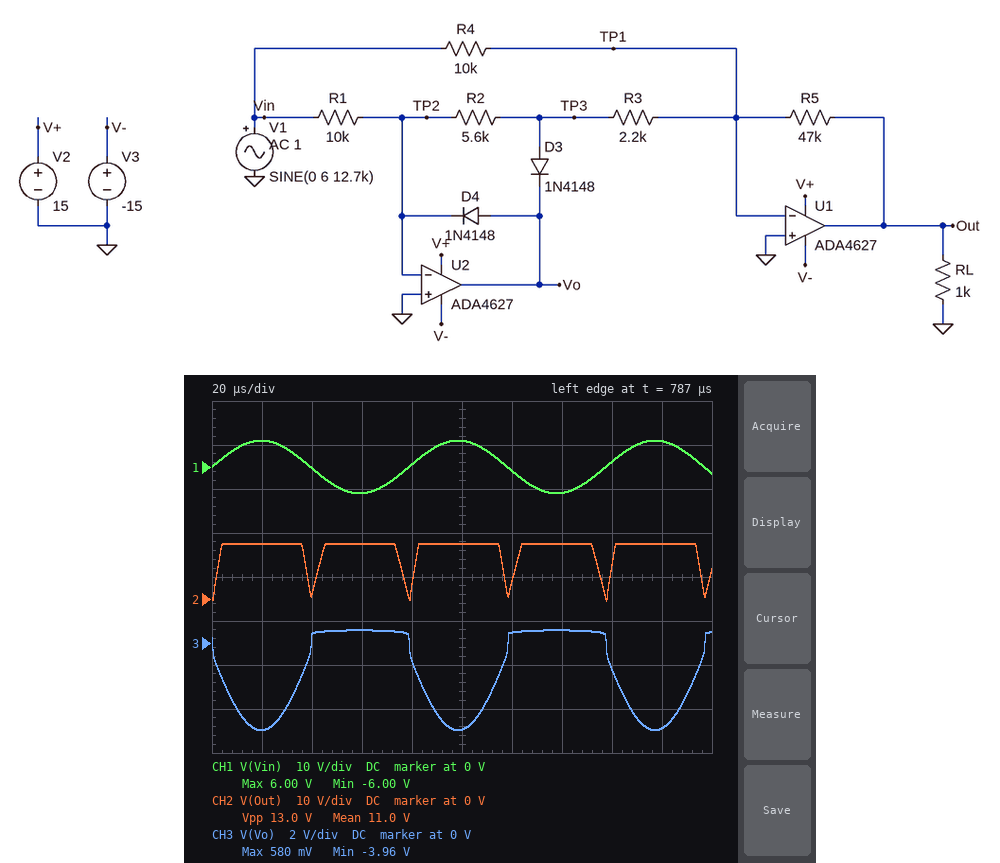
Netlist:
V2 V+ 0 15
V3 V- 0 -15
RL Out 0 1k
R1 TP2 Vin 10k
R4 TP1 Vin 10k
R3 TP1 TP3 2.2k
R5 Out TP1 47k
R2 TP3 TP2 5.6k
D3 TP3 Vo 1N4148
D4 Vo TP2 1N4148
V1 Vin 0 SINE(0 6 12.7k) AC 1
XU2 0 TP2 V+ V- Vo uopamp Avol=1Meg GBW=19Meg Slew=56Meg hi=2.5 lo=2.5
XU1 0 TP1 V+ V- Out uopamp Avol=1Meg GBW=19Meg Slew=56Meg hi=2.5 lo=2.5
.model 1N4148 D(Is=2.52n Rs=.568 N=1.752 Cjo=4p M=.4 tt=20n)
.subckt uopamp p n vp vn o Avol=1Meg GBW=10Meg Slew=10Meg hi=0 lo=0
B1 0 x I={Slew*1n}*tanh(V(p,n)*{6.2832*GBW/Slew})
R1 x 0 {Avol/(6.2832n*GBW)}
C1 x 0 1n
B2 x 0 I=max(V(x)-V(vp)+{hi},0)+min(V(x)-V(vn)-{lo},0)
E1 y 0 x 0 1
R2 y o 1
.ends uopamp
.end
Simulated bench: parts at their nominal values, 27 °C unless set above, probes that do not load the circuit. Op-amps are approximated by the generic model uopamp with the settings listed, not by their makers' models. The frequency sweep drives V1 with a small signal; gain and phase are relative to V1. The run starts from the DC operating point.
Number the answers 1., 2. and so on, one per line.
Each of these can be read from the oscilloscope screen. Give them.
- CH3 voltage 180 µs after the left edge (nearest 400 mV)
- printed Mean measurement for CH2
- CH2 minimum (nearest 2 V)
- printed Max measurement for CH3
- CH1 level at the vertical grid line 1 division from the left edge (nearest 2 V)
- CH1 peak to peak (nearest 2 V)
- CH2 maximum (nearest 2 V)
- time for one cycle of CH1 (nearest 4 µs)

1. -4.0 V
2. 11.0 V
3. 0 V
4. 580 mV
5. 6 V
6. 12 V
7. 12 V
8. 80 µs
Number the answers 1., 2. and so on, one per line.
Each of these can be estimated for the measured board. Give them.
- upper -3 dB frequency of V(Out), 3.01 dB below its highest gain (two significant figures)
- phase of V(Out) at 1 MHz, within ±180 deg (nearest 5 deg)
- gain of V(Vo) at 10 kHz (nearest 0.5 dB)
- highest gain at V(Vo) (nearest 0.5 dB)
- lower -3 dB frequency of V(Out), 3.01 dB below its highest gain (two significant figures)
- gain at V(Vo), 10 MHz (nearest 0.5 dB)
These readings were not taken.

1. 1.5 MHz
2. 145 deg
3. 47.0 dB
4. 63.0 dB
5. 870 Hz
6. -11.0 dB
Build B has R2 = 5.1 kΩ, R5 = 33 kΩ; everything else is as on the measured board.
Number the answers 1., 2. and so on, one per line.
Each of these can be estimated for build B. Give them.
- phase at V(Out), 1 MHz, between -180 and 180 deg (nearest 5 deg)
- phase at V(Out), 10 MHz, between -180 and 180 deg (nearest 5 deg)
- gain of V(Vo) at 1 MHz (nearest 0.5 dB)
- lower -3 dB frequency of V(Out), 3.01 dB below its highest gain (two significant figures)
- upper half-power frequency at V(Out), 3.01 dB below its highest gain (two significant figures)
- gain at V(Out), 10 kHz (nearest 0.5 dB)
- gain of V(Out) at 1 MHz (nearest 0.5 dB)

1. 155 deg
2. 95 deg
3. 7.5 dB
4. 830 Hz
5. 2.1 MHz
6. 8.0 dB
7. 7.0 dB
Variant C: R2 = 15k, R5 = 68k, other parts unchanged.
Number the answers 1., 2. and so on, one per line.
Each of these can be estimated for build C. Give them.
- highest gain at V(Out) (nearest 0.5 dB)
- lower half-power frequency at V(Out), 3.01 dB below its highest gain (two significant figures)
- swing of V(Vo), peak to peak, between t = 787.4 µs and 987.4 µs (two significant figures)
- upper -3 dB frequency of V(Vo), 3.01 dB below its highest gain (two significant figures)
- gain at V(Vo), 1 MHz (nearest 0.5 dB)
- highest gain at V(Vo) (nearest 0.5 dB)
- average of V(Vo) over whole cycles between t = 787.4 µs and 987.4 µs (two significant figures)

1. 10.5 dB
2. 1.3 kHz
3. 10 V
4. 1.7 kHz
5. 9.0 dB
6. 64.0 dB
7. -2.9 V
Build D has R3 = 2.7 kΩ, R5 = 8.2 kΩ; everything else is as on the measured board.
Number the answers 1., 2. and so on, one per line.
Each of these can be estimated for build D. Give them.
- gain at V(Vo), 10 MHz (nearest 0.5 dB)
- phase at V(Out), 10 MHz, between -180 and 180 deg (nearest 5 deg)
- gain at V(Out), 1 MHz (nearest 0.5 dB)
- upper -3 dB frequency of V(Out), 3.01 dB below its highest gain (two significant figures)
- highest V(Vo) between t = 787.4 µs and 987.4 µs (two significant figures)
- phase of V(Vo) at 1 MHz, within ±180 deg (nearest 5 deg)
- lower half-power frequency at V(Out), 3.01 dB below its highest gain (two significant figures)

1. -11.5 dB
2. 120 deg
3. -4.0 dB
4. 7.7 MHz
5. 560 mV
6. 90 deg
7. 660 Hz
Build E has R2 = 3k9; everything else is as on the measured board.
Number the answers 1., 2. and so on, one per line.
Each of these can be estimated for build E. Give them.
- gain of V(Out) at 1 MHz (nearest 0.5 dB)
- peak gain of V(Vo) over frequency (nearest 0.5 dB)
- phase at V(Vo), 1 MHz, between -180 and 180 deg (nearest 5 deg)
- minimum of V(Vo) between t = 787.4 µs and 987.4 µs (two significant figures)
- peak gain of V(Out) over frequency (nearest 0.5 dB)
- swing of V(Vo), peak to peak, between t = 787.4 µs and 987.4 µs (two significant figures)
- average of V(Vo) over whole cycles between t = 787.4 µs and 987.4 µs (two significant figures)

1. 10.0 dB
2. 62.5 dB
3. 100 deg
4. -2.9 V
5. 12.0 dB
6. 3.5 V
7. -760 mV
